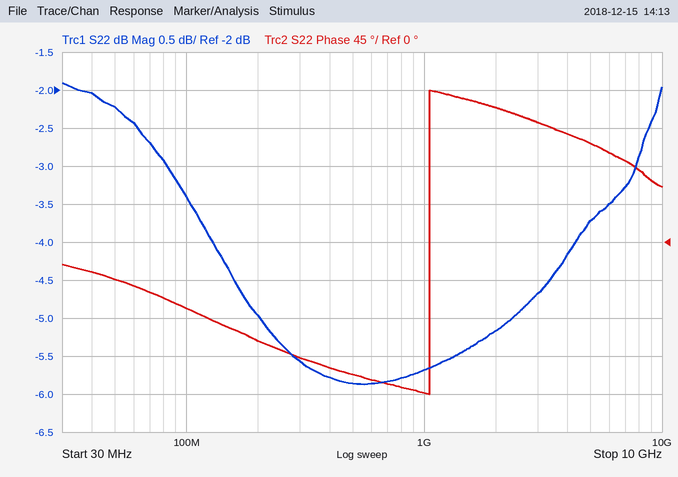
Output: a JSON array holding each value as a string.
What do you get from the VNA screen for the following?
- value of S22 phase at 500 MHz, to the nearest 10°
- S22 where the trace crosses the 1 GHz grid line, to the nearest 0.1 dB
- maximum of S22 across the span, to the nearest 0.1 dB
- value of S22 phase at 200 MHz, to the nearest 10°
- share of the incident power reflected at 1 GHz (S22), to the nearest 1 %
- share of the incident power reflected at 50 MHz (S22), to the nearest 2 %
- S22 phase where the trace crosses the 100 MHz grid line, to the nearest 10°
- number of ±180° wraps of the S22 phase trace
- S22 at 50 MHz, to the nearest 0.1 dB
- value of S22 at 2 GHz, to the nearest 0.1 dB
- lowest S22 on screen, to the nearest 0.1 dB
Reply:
["-160°", "-5.7 dB", "-1.9 dB", "-120°", "27 %", "60 %", "-80°", "1", "-2.2 dB", "-5.2 dB", "-5.9 dB"]
